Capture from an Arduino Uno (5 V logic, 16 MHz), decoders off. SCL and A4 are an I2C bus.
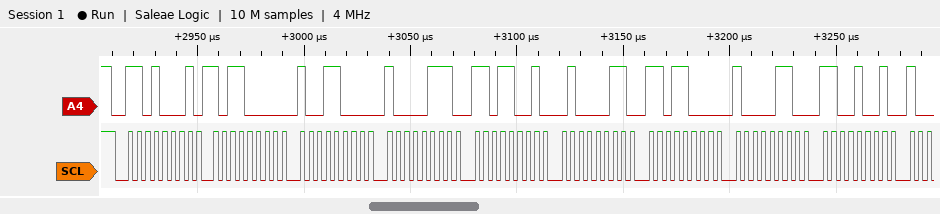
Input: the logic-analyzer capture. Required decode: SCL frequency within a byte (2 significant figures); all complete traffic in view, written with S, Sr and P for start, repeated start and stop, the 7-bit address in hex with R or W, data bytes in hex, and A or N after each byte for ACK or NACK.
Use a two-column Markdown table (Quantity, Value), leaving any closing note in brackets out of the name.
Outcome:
| Quantity | Value |
|---|---|
| SCL frequency within a byte | 250 kHz |
| all complete traffic in view, written with S, Sr and P for start, repeated start and stop, the 7-bit address in hex with R or W, data bytes in hex, and A or N after each byte for ACK or NACK | S 68R A B0 A 98 A 87 A D9 A 43 A D8 A 86 A C9 A |
